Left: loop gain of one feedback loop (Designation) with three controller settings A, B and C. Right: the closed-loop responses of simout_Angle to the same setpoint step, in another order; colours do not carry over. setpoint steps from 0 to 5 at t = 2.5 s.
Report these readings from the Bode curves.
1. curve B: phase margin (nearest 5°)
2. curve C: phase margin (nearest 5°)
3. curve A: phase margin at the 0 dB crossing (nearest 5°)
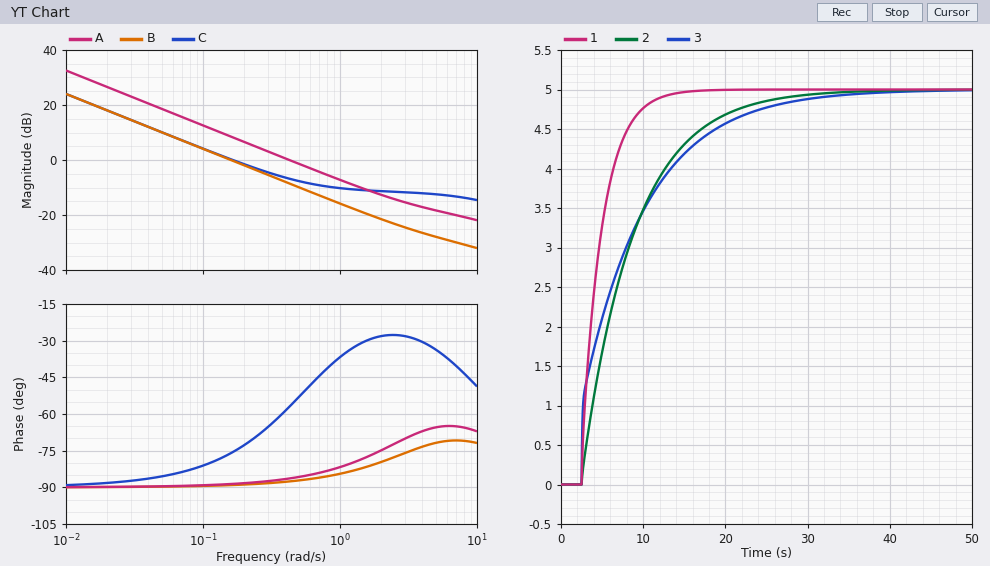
90°
105°
95°
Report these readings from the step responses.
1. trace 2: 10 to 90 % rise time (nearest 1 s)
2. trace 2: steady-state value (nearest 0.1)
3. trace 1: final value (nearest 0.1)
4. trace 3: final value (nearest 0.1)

14 s
5.0
5.0
5.0
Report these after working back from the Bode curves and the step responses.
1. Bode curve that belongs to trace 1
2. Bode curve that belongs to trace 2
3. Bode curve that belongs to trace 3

A
B
C
